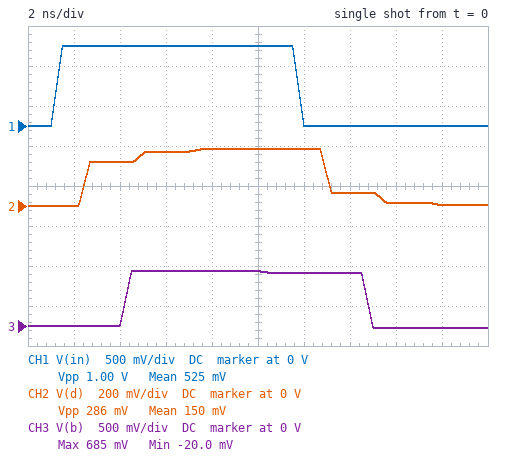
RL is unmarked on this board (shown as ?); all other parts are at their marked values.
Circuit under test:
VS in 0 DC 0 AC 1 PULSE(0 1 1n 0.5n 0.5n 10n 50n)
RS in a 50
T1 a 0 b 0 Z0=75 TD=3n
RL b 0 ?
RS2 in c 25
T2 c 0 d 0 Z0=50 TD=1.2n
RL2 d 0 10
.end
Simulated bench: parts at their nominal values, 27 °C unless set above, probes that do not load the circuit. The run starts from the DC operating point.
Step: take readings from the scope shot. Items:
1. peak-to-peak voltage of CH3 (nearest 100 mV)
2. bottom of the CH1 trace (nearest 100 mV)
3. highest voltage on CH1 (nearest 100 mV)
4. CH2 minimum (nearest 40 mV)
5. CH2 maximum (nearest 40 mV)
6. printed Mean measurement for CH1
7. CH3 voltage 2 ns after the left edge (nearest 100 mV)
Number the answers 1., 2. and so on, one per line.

1. 700 mV
2. 0 V
3. 1.0 V
4. 0 V
5. 280 mV
6. 525 mV
7. 0 V
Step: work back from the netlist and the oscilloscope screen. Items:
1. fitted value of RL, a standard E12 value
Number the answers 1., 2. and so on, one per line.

1. 100 Ω
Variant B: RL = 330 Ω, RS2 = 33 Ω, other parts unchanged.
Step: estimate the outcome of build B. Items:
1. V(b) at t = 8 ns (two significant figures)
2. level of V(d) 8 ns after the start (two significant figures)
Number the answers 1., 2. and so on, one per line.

1. 980 mV
2. 230 mV
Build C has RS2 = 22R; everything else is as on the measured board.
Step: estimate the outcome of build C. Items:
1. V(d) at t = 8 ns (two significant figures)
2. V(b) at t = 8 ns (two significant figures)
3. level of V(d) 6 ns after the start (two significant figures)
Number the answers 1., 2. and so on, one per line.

1. 310 mV
2. 690 mV
3. 290 mV
